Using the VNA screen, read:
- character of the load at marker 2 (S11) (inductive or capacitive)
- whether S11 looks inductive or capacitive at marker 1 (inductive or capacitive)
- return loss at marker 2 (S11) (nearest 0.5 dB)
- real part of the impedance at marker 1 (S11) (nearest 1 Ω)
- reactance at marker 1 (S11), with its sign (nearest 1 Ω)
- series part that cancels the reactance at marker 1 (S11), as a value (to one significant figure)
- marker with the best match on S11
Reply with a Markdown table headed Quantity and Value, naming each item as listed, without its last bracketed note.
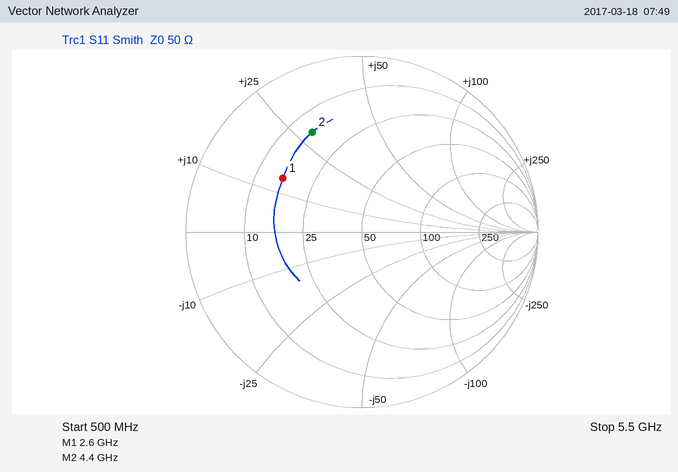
| Quantity | Value |
|---|---|
| character of the load at marker 2 (S11) | inductive |
| whether S11 looks inductive or capacitive at marker 1 | inductive |
| return loss at marker 2 (S11) | 4.0 dB |
| real part of the impedance at marker 1 (S11) | 16 Ω |
| reactance at marker 1 (S11), with its sign | +14 Ω |
| series part that cancels the reactance at marker 1 (S11), as a value | 4 pF |
| marker with the best match on S11 | marker 1 |
